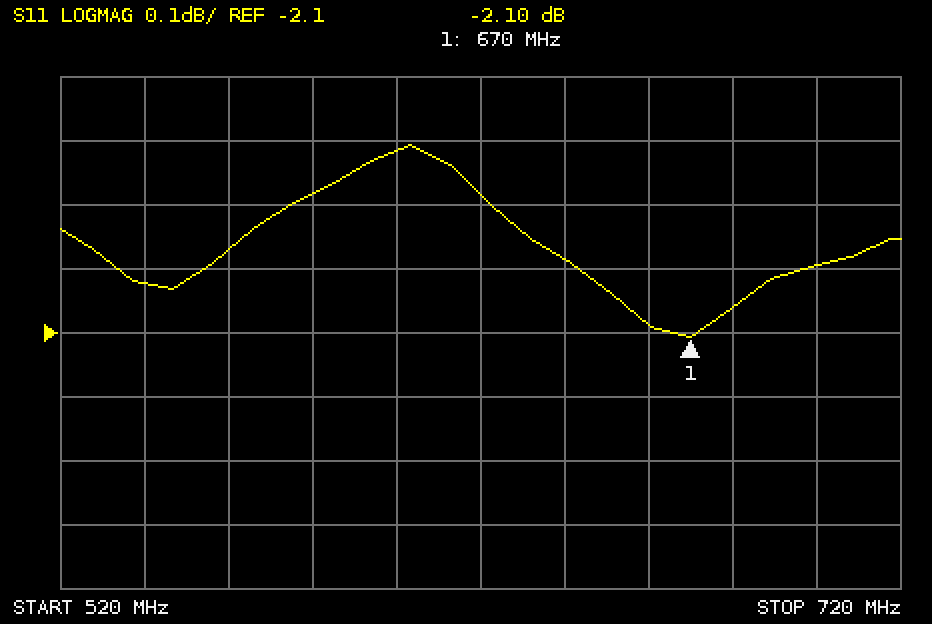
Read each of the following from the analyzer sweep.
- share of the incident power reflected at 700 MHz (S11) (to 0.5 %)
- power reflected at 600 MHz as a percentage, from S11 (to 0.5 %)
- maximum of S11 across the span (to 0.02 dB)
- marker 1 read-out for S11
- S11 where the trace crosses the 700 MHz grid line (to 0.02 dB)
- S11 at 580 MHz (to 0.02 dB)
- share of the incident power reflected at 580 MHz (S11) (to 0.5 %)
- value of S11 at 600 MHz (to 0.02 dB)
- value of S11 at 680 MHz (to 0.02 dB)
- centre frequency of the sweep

63.0 %
66.0 %
-1.80 dB
-2.10 dB
-2.00 dB
-1.88 dB
65.0 %
-1.82 dB
-2.06 dB
620 MHz
